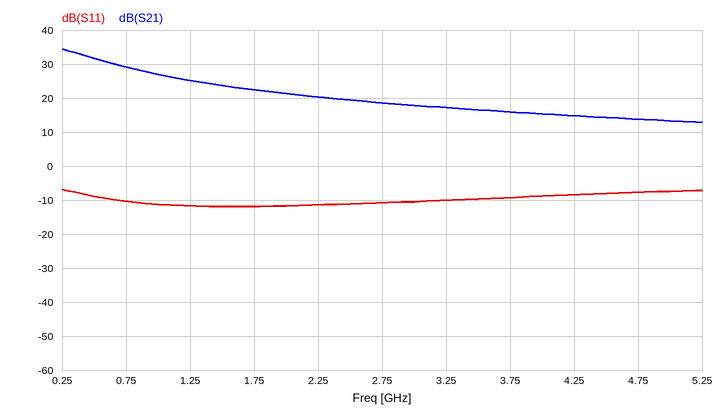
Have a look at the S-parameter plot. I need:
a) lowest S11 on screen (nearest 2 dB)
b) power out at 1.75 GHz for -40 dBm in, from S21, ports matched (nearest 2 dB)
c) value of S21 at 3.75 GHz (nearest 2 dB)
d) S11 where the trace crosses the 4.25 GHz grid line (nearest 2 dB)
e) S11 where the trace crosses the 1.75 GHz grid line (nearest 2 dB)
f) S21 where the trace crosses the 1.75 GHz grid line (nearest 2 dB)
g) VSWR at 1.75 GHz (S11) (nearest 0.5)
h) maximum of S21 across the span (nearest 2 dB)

-12 dB
-18 dBm
16 dB
-8 dB
-12 dB
22 dB
1.5
34 dB
